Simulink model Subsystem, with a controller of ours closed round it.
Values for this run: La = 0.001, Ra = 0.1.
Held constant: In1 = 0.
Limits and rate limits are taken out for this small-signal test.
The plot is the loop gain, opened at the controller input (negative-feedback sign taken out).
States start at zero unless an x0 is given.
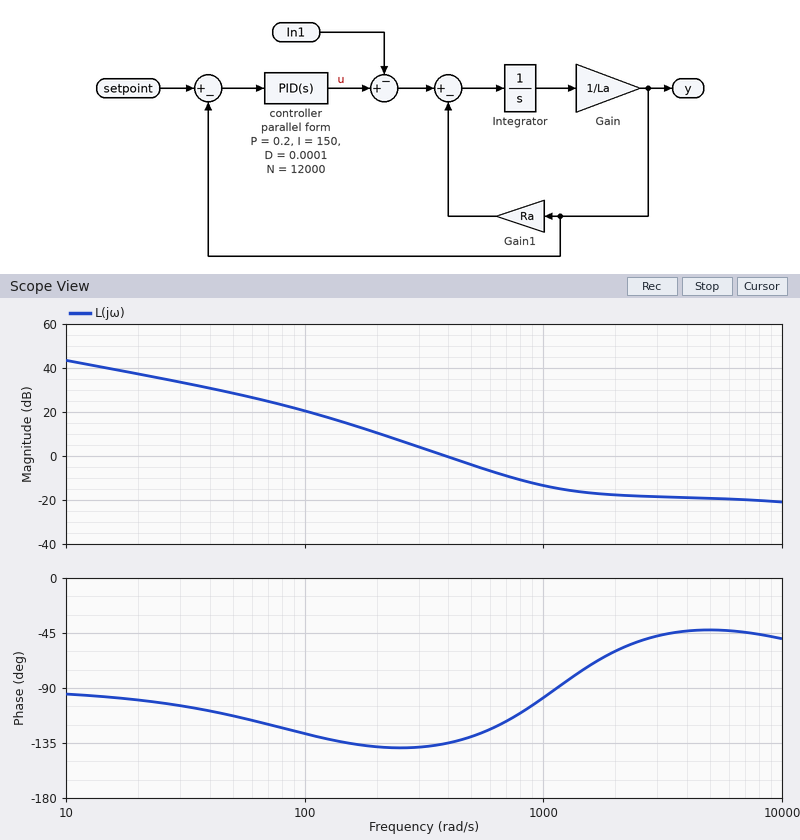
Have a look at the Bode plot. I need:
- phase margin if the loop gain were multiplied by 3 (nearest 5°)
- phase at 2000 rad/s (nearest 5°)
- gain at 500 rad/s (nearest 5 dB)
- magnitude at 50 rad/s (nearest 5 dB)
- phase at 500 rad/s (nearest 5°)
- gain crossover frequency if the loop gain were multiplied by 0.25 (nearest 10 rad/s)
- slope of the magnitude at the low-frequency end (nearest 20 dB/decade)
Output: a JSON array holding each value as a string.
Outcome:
["65°", "-60°", "-5 dB", "30 dB", "-130°", "180 rad/s", "-20 dB/decade"]
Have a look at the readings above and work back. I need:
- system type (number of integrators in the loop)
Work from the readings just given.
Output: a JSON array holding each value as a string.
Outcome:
["1"]
